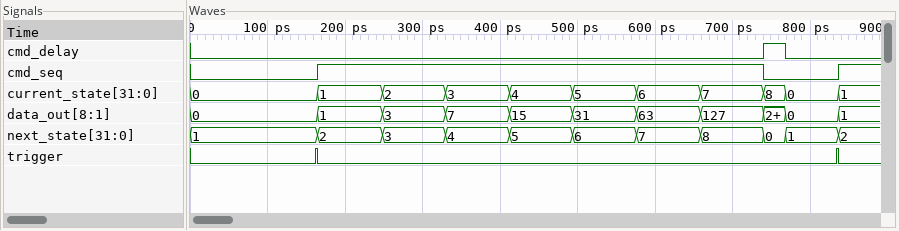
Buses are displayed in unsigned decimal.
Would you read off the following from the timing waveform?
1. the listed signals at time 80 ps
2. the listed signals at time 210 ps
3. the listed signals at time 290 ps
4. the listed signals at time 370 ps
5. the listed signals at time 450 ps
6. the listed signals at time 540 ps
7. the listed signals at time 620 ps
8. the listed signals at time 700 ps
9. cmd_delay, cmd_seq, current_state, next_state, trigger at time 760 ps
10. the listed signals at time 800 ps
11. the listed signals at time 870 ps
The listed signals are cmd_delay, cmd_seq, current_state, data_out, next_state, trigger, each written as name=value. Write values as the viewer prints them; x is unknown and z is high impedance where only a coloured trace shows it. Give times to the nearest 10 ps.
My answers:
cmd_delay=0, cmd_seq=0, current_state=0, data_out=0, next_state=1, trigger=0
cmd_delay=0, cmd_seq=1, current_state=1, data_out=1, next_state=2, trigger=0
cmd_delay=0, cmd_seq=1, current_state=2, data_out=3, next_state=3, trigger=0
cmd_delay=0, cmd_seq=1, current_state=3, data_out=7, next_state=4, trigger=0
cmd_delay=0, cmd_seq=1, current_state=4, data_out=15, next_state=5, trigger=0
cmd_delay=0, cmd_seq=1, current_state=5, data_out=31, next_state=6, trigger=0
cmd_delay=0, cmd_seq=1, current_state=6, data_out=63, next_state=7, trigger=0
cmd_delay=0, cmd_seq=1, current_state=7, data_out=127, next_state=8, trigger=0
cmd_delay=1, cmd_seq=0, current_state=8, next_state=0, trigger=0
cmd_delay=0, cmd_seq=0, current_state=0, data_out=0, next_state=1, trigger=0
cmd_delay=0, cmd_seq=1, current_state=1, data_out=1, next_state=2, trigger=0
